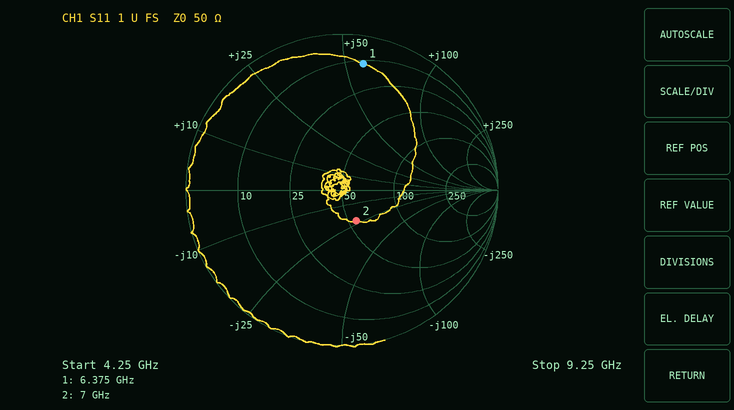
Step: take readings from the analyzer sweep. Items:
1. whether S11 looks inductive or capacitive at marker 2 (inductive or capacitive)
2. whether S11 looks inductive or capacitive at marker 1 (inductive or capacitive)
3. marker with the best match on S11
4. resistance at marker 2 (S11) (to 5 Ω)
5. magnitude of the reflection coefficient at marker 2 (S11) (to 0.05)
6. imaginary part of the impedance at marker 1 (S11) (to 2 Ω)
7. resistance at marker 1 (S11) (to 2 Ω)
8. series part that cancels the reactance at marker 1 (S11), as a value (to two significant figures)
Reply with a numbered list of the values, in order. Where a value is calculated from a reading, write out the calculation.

1. capacitive
2. inductive
3. marker 2
4. 55 Ω
5. 0.20
6. +58 Ω
7. 12 Ω
8. C = 1/(2π × 6.375 GHz × 58 Ω) ≈ 430 fF
